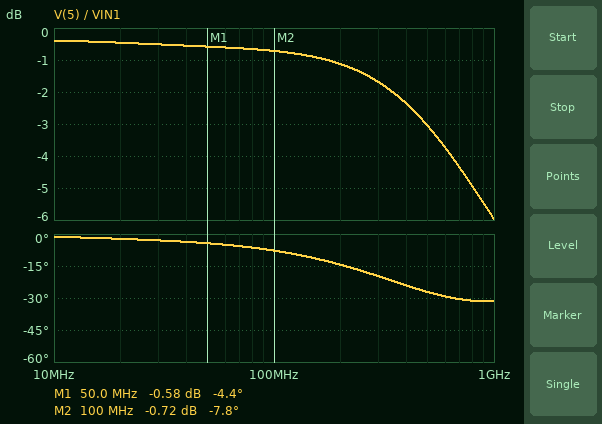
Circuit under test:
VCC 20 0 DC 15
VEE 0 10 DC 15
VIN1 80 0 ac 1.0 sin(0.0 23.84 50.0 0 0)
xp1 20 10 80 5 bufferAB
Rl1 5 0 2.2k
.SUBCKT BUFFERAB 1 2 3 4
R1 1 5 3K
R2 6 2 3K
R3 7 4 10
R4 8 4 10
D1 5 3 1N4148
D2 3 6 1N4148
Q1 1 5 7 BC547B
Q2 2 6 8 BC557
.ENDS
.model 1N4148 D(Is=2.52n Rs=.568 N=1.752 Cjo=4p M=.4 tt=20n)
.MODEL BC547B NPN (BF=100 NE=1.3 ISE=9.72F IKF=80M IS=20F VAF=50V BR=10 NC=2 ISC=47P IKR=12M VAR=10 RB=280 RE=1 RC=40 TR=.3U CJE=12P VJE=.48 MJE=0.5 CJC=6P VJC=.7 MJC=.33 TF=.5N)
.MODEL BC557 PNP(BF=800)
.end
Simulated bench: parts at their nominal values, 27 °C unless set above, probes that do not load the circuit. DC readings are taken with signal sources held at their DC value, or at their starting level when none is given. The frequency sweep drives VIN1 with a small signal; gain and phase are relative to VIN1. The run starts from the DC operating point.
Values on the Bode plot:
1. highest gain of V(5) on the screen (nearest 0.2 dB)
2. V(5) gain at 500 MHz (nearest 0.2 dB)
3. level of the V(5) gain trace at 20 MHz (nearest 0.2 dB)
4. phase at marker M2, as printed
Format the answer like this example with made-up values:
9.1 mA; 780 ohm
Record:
-0.4 dB; -3.0 dB; -0.4 dB; -7.8 deg
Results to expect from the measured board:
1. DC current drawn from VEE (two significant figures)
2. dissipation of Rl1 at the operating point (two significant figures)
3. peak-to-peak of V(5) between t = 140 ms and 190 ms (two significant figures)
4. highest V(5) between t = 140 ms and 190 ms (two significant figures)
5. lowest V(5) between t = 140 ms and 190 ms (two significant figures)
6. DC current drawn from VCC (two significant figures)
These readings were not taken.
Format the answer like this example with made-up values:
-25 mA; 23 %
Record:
4.9 mA; 2.1 µW; 28 V; 14 V; -14 V; 5.0 mA
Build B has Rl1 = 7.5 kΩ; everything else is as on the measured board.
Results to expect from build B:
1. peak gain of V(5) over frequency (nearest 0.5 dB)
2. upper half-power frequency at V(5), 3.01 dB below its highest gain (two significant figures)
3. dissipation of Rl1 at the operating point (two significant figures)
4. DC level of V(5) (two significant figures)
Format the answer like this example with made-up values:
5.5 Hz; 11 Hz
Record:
0 dB; 560 MHz; 660 nW; 70 mV
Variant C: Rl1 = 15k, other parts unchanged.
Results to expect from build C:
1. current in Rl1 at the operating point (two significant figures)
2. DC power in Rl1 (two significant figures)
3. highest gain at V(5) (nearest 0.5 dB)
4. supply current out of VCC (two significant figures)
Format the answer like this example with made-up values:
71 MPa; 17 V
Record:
4.7 µA; 330 nW; 0 dB; 4.9 mA
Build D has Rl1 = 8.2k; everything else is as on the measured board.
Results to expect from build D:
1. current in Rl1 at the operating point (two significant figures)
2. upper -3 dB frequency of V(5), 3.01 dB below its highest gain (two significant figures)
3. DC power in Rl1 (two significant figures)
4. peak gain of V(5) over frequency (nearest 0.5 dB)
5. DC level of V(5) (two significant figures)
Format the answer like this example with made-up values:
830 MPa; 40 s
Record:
8.6 µA; 560 MHz; 600 nW; 0 dB; 70 mV
